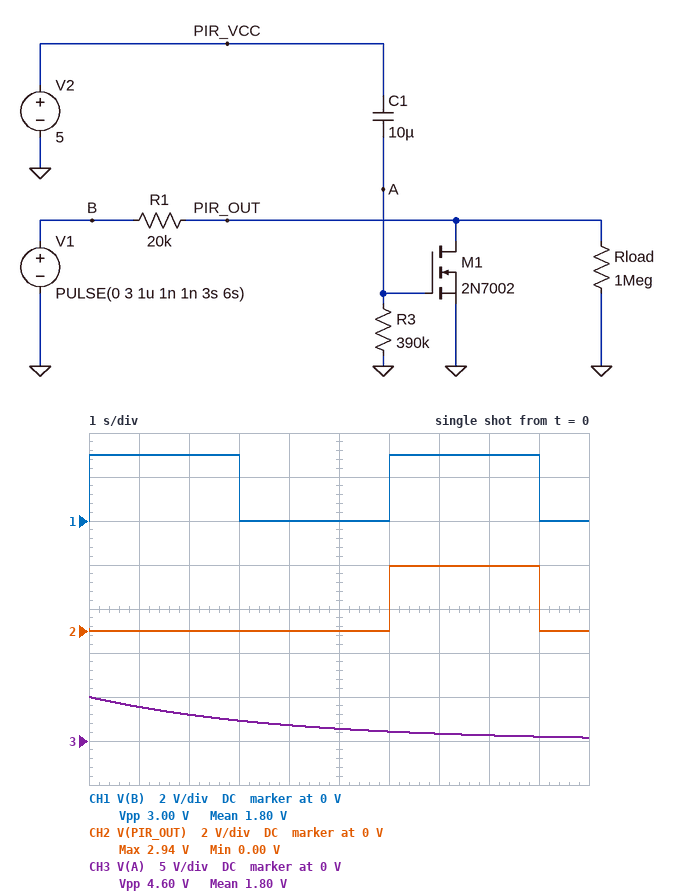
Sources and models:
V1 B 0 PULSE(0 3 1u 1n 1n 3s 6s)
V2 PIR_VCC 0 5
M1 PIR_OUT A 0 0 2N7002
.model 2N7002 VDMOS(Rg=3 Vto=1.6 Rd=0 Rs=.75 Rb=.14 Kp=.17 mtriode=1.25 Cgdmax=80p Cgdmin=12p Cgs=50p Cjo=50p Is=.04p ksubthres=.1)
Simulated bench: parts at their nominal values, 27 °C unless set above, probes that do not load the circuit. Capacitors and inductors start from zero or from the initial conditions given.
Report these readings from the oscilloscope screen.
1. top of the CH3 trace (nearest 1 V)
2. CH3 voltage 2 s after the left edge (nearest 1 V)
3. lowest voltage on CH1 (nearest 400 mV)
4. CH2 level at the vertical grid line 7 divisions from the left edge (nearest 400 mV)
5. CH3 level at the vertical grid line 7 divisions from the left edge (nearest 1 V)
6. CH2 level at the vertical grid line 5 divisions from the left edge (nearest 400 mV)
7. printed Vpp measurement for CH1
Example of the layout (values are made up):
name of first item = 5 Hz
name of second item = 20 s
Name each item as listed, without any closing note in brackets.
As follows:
top of the CH3 trace = 5 V
CH3 voltage 2 s after the left edge = 3 V
lowest voltage on CH1 = 0 V
CH2 level at the vertical grid line 7 divisions from the left edge = 2.8 V
CH3 level at the vertical grid line 7 divisions from the left edge = 1 V
CH2 level at the vertical grid line 5 divisions from the left edge = 0 V
printed Vpp measurement for CH1 = 3.00 V
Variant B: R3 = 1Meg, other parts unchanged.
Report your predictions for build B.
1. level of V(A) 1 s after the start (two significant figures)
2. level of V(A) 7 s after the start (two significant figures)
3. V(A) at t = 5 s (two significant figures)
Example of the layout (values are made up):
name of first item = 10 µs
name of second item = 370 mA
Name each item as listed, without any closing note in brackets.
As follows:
level of V(A) 1 s after the start = 4.5 V
level of V(A) 7 s after the start = 2.5 V
V(A) at t = 5 s = 3.0 V
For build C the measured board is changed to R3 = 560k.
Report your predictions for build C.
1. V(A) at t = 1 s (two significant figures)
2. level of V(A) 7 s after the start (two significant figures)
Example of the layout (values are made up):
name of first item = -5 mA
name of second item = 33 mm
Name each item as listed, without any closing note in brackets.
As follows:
V(A) at t = 1 s = 4.2 V
level of V(A) 7 s after the start = 1.4 V
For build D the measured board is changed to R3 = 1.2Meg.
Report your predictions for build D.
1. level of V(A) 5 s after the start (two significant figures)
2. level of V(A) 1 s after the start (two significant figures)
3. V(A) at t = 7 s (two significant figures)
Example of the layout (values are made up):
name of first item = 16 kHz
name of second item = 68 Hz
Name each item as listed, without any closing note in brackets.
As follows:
level of V(A) 5 s after the start = 3.3 V
level of V(A) 1 s after the start = 4.6 V
V(A) at t = 7 s = 2.8 V
